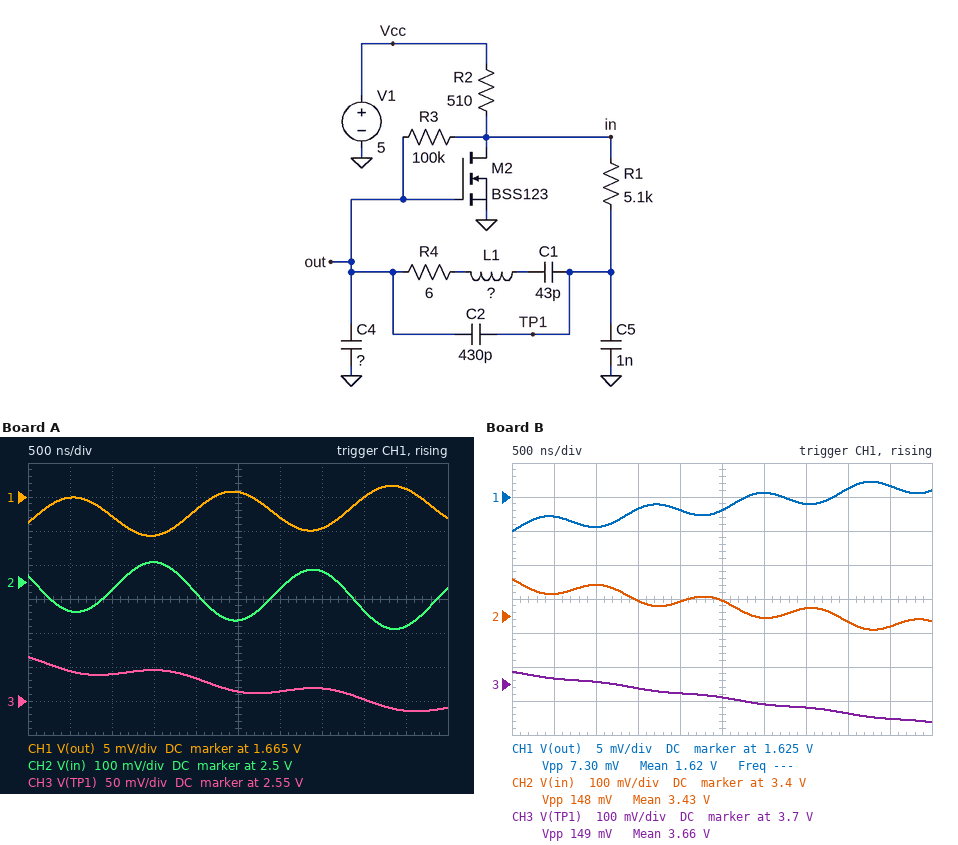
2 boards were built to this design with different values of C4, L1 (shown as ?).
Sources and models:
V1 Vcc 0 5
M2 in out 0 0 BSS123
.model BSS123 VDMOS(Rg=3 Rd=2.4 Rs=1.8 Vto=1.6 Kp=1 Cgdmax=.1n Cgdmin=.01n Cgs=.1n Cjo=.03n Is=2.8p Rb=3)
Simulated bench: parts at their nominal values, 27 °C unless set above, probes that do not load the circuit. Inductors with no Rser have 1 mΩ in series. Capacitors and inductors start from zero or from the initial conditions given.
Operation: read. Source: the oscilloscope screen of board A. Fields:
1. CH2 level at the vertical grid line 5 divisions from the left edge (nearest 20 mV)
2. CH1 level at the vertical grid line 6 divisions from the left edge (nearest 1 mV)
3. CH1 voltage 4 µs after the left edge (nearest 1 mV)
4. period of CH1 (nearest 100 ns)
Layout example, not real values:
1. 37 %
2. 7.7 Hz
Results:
1. 2.38 V
2. 1.662 V
3. 1.665 V
4. 1.8 µs
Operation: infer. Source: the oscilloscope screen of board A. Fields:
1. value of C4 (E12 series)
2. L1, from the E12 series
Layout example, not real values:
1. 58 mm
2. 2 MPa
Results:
1. 1.5 nF
2. 2.2 mH
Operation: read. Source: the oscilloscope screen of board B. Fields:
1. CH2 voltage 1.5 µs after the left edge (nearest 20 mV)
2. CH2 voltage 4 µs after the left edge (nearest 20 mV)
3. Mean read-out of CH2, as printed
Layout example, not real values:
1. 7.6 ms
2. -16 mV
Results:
1. 3.44 V
2. 3.38 V
3. 3.43 V
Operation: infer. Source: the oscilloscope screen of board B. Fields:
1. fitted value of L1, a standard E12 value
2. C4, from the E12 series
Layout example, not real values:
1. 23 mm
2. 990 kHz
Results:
1. 1 mH
2. 1.8 nF
